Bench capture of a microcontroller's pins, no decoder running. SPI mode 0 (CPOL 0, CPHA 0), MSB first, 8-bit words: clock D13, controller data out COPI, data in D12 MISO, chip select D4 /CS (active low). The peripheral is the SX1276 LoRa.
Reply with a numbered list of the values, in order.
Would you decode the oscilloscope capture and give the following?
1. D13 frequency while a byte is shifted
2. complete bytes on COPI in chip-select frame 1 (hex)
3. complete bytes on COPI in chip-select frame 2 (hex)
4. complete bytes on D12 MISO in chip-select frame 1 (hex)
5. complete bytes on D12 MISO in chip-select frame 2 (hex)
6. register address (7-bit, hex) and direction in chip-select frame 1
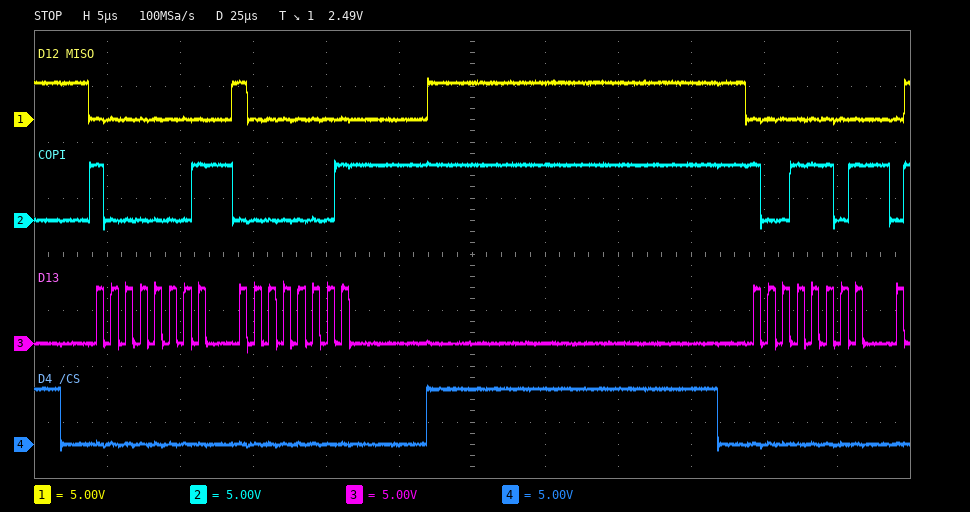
1. 1 MHz
2. 81 01
3. 9D
4. 00 80
5. 00
6. 0x01 write
